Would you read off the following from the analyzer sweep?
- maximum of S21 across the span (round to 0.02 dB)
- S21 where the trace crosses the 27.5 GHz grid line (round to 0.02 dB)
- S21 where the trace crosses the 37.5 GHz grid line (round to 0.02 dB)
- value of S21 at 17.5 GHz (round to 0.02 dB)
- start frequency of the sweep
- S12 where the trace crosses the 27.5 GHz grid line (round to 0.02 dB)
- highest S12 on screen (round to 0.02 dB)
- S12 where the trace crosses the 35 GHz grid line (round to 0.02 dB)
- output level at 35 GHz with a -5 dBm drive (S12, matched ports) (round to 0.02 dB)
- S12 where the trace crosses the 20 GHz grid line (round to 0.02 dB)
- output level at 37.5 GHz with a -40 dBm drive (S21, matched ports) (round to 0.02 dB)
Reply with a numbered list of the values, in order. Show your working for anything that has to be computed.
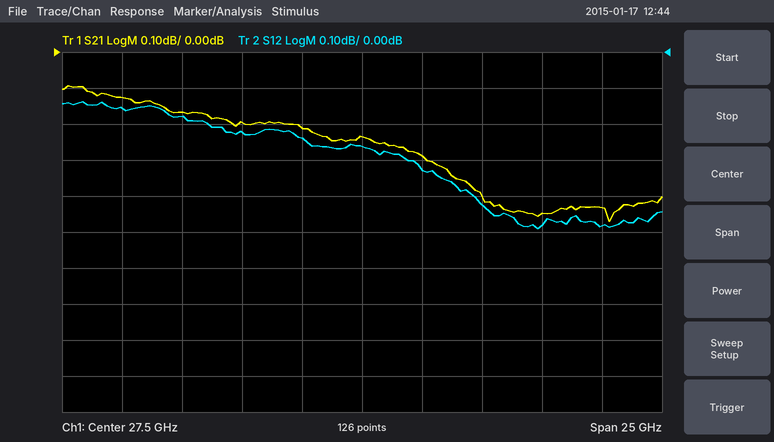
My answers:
1. -0.10 dB
2. -0.24 dB
3. -0.44 dB
4. -0.12 dB
5. 15 GHz
6. -0.26 dB
7. -0.14 dB
8. -0.48 dB
9. -5 dBm + (-0.48 dB) = -5.48 dBm
10. -0.18 dB
11. -40 dBm + (-0.44 dB) = -40.44 dBm
